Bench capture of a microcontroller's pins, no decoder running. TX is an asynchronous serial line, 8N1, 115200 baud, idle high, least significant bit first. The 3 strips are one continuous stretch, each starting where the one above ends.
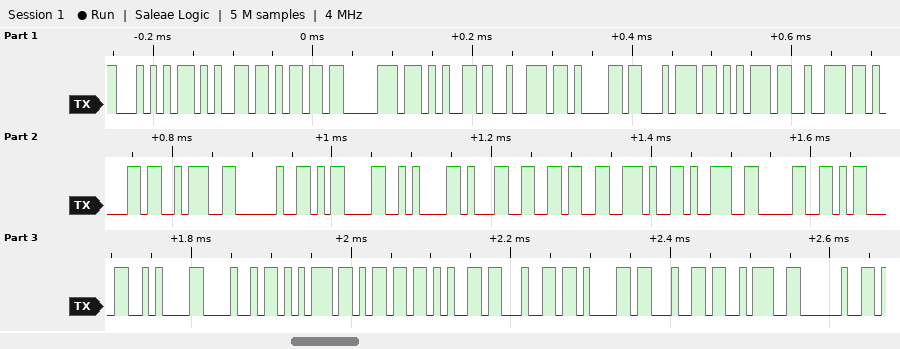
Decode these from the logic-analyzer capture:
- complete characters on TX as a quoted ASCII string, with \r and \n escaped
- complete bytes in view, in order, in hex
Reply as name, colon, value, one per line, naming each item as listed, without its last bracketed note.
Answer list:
complete characters on TX as a quoted ASCII string, with \r and \n escaped: "Temperatura: \r\n16.90\r\nHumedad: "
complete bytes in view, in order, in hex: 54 65 6D 70 65 72 61 74 75 72 61 3A 20 0D 0A 31 36 2E 39 30 0D 0A 48 75 6D 65 64 61 64 3A 20
